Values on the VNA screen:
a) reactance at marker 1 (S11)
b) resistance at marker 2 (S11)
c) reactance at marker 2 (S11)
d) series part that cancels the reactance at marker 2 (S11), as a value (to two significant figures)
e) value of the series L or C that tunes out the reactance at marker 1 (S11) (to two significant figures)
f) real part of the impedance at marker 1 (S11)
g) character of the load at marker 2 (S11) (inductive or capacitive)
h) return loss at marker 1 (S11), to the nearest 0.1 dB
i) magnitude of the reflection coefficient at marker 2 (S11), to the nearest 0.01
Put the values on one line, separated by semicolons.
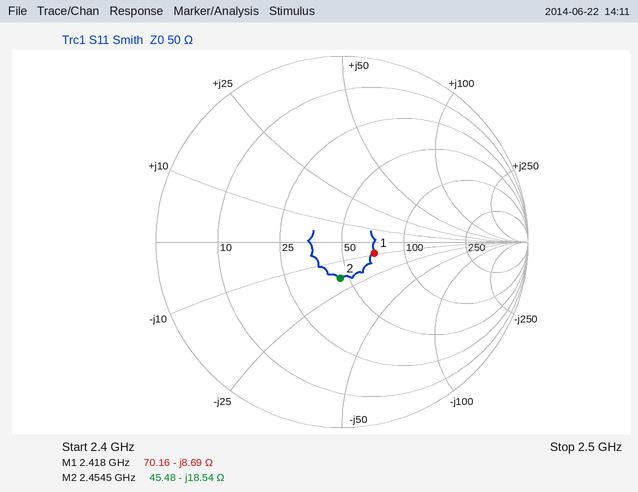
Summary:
-8.69 Ω; 45.48 Ω; -18.54 Ω; 1.2 nH; 570 pH; 70.16 Ω; capacitive; 14.8 dB; 0.20
